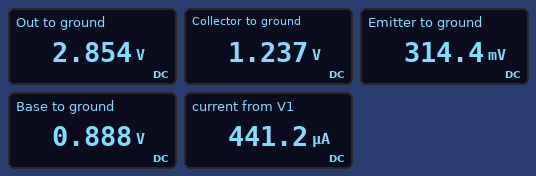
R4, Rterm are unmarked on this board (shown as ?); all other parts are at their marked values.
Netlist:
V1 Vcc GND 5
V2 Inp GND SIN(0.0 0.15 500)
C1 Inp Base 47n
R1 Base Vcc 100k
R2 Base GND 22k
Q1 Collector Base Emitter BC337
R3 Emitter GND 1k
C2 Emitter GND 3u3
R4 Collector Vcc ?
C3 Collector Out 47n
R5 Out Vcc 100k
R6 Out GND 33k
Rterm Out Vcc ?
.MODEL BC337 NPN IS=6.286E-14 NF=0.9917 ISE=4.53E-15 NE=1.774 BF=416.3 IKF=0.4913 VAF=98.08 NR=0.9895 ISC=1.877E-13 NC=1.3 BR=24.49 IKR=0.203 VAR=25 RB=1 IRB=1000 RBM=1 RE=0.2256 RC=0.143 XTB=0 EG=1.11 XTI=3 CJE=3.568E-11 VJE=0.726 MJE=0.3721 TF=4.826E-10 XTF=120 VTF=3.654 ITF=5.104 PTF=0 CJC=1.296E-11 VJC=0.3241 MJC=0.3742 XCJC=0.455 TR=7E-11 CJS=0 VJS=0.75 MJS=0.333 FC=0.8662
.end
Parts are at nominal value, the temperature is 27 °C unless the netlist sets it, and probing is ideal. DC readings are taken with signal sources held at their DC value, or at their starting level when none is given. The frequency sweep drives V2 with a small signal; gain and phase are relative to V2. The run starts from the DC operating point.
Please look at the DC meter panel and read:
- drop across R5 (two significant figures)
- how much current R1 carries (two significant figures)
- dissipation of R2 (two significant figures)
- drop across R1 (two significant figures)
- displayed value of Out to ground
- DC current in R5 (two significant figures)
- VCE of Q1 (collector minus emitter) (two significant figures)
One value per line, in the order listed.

2.1 V
41 µA
36 µW
4.1 V
2.854 V
21 µA
920 mV
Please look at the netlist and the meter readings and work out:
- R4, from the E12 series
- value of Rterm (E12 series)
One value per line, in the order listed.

12 kΩ
33 kΩ
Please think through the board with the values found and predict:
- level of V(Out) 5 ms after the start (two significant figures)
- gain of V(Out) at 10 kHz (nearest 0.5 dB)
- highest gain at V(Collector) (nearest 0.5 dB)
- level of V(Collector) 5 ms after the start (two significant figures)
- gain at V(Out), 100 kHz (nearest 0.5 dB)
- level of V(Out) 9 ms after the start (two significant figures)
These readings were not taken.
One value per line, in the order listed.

4.5 V
37.5 dB
37.5 dB
3.5 V
37.5 dB
4.5 V
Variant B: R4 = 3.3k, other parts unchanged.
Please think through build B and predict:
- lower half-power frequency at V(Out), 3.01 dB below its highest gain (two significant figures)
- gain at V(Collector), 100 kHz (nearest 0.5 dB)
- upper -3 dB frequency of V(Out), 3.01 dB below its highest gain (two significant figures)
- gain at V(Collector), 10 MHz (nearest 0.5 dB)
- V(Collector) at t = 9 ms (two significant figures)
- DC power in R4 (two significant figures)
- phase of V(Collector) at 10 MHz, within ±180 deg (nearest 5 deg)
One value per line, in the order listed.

830 Hz
30.0 dB
11 MHz
27.5 dB
4.8 V
330 µW
135 deg
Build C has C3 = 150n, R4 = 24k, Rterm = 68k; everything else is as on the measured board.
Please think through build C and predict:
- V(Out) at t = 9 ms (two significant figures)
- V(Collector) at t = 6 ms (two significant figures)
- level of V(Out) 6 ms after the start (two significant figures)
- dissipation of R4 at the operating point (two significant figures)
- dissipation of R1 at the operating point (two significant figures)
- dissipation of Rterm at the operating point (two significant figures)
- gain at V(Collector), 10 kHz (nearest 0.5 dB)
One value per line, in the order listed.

3.7 V
180 mV
1.4 V
950 µW
180 µW
110 µW
5.0 dB
